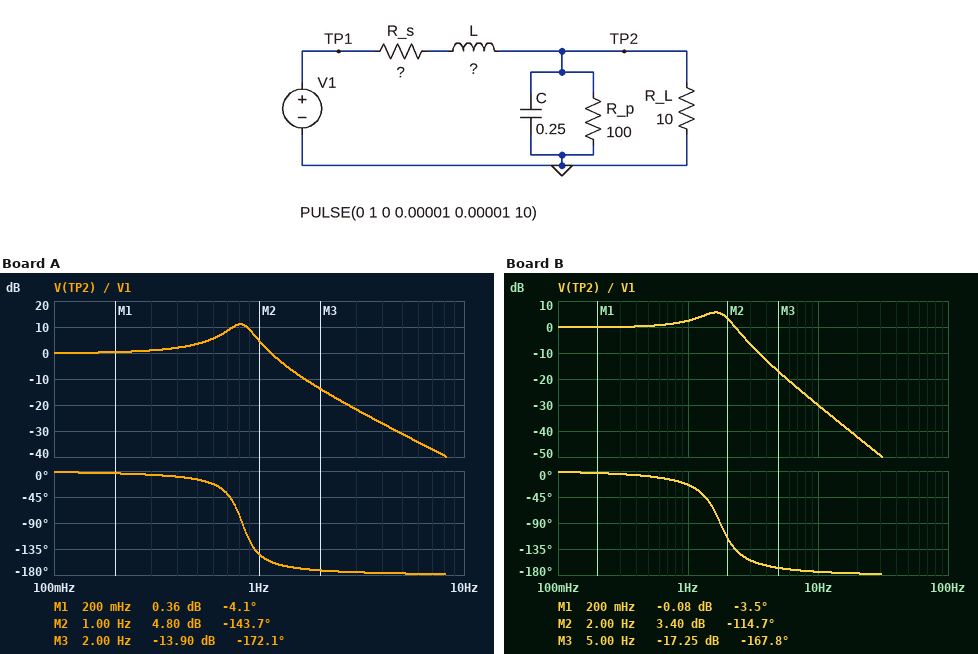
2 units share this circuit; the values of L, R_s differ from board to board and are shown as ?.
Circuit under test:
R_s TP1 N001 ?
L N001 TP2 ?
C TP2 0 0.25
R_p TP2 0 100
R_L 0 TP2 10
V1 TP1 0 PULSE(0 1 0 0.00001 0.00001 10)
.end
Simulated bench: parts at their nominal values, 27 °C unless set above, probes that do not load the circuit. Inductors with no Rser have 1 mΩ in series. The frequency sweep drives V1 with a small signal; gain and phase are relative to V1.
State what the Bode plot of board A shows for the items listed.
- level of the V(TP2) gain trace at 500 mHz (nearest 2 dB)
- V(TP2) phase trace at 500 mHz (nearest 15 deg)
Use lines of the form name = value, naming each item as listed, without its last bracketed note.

level of the V(TP2) gain trace at 500 mHz = 4 dB
V(TP2) phase trace at 500 mHz = -15 deg
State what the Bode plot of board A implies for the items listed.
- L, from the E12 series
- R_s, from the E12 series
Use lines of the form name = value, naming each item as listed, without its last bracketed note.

L, from the E12 series = 150 mH
R_s, from the E12 series = 0.15 Ω
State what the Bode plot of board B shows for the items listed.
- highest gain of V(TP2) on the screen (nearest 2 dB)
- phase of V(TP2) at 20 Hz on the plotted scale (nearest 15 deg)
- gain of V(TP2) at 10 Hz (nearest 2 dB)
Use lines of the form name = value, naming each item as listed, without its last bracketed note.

highest gain of V(TP2) on the screen = 6 dB
phase of V(TP2) at 20 Hz on the plotted scale = -180 deg
gain of V(TP2) at 10 Hz = -30 dB
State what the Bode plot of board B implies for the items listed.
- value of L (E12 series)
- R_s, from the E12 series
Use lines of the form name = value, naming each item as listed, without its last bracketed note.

value of L = 33 mH
R_s, from the E12 series = 0.18 Ω
